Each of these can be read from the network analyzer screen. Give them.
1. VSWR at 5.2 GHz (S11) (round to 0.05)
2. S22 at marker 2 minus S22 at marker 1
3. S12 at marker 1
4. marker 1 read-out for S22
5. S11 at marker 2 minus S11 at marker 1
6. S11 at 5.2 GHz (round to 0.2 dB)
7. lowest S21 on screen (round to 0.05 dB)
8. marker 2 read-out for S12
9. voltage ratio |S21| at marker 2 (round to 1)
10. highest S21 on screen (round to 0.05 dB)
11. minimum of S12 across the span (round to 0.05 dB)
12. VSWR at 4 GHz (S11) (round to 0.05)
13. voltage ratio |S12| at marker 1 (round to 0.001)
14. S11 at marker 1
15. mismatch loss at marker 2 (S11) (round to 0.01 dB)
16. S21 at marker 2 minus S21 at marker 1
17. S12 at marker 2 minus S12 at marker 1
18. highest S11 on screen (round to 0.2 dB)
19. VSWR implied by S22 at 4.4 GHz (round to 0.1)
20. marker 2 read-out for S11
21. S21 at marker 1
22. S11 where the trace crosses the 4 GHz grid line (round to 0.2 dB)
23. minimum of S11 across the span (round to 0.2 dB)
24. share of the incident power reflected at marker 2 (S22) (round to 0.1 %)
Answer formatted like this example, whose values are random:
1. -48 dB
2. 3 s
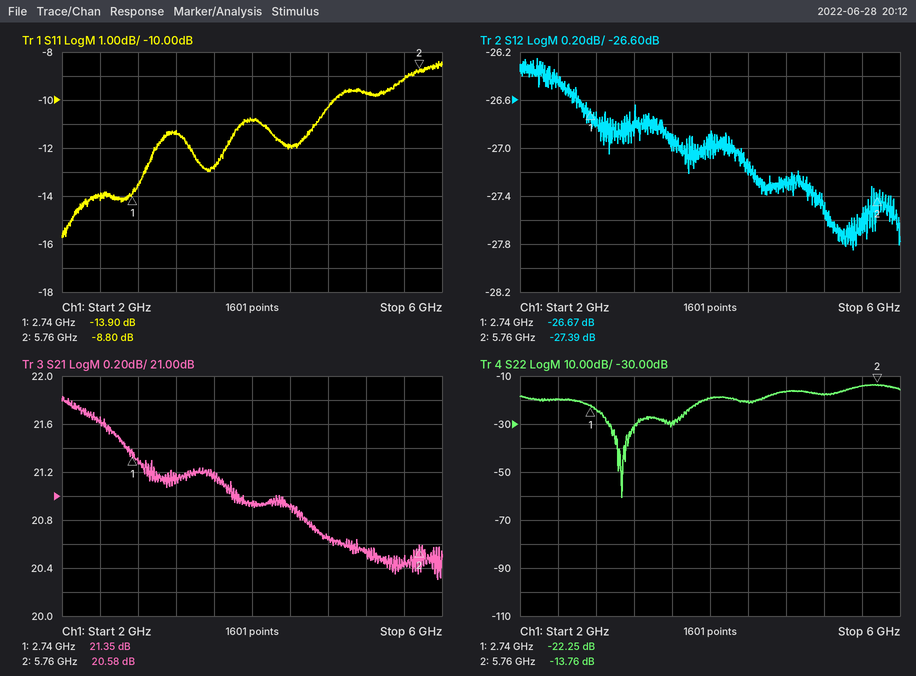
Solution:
1. 1.95
2. 8.49 dB
3. -26.67 dB
4. -22.25 dB
5. 5.10 dB
6. -9.8 dB
7. 20.30 dB
8. -27.39 dB
9. 11
10. 21.85 dB
11. -27.85 dB
12. 1.80
13. 0.046
14. -13.90 dB
15. 0.61 dB
16. -0.77 dB
17. -0.72 dB
18. -8.4 dB
19. 1.2
20. -8.80 dB
21. 21.35 dB
22. -10.8 dB
23. -15.8 dB
24. 4.2 %
